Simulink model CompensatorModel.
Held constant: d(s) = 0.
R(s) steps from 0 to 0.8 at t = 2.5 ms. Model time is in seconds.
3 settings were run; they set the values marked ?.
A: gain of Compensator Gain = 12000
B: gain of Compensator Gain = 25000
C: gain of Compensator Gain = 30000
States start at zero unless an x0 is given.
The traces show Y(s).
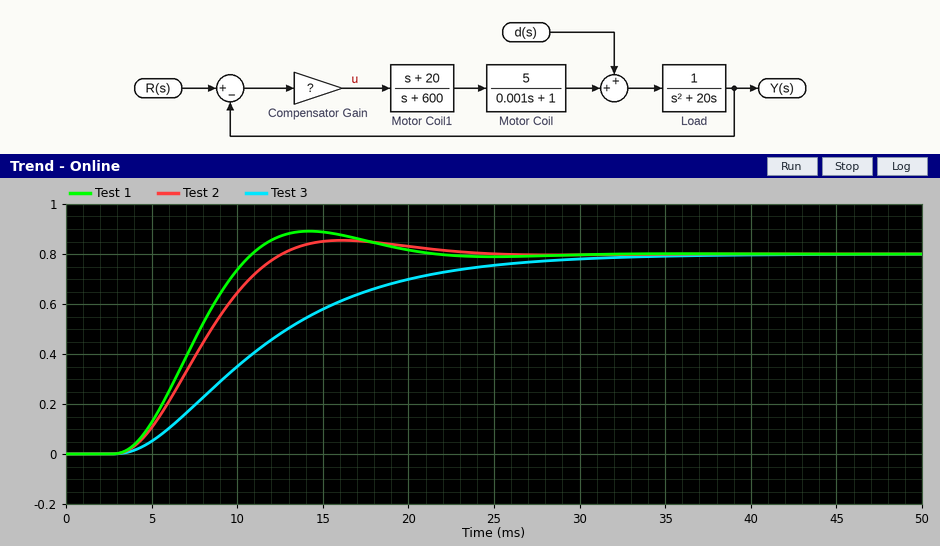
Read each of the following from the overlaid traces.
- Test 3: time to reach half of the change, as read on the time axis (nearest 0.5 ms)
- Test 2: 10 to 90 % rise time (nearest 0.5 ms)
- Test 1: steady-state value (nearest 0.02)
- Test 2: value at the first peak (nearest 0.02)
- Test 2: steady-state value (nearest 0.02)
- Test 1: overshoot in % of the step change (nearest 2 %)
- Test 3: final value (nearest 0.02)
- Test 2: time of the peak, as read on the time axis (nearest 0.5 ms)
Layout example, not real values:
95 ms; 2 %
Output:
11.0 ms; 6.5 ms; 0.80; 0.86; 0.80; 12 %; 0.80; 16.0 ms
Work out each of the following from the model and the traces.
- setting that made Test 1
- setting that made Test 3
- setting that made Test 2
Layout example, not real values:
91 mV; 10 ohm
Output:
C; A; B
